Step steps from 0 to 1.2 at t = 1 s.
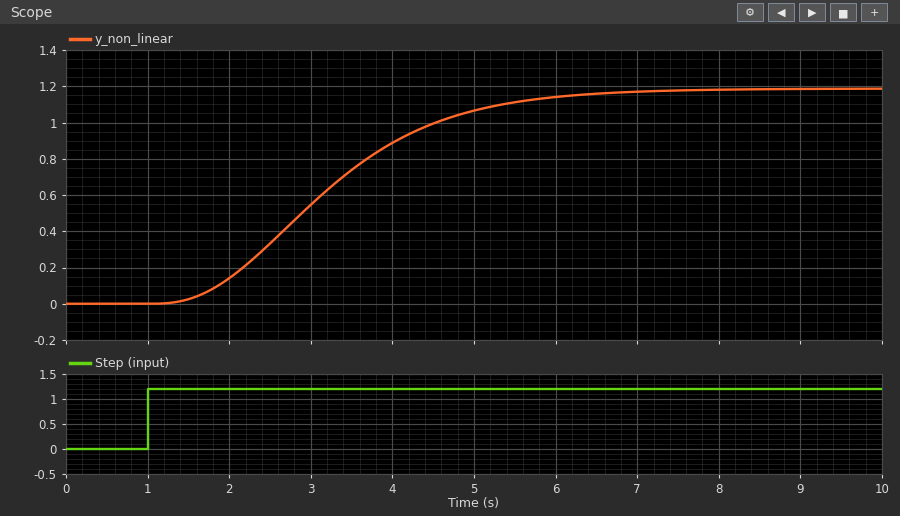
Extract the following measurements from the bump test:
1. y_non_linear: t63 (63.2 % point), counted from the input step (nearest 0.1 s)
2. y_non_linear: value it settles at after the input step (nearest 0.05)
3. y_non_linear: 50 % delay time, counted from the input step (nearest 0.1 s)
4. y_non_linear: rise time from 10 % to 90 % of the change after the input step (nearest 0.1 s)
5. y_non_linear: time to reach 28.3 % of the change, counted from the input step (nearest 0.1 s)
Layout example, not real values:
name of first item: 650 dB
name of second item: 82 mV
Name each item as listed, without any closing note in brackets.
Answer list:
y_non_linear: t63 (63.2 % point), counted from the input step: 2.5 s
y_non_linear: value it settles at after the input step: 1.20
y_non_linear: 50 % delay time, counted from the input step: 2.1 s
y_non_linear: rise time from 10 % to 90 % of the change after the input step: 3.1 s
y_non_linear: time to reach 28.3 % of the change, counted from the input step: 1.5 s
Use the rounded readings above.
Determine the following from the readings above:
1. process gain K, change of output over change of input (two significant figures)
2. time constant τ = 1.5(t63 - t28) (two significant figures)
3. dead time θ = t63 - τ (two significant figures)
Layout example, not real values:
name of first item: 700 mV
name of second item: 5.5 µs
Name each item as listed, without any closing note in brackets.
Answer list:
process gain K, change of output over change of input: 1.0
time constant τ = 1.5(t63 - t28): 1.5 s
dead time θ = t63 - τ: 1.0 s
